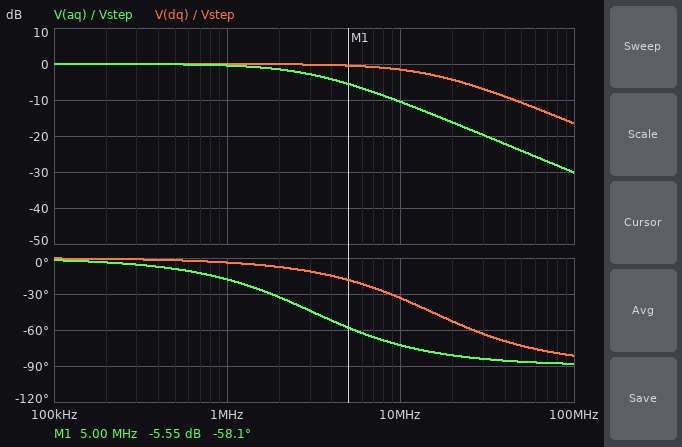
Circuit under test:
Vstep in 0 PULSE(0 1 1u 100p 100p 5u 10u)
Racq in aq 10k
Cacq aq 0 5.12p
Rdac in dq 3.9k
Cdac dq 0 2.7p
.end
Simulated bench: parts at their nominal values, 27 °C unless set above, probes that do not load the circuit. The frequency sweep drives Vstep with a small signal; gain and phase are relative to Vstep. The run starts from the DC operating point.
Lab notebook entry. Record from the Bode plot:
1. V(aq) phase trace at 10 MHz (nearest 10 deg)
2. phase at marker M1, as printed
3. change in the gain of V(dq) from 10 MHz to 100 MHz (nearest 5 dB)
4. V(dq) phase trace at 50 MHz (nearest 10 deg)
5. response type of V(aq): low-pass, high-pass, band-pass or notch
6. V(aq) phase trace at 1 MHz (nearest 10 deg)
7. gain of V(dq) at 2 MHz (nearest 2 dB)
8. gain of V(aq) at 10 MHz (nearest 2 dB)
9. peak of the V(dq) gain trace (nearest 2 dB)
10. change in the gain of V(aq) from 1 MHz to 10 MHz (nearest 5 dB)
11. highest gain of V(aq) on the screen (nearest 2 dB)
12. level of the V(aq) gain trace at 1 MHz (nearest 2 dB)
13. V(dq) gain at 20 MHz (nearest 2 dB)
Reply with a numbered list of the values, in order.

1. -70 deg
2. -58.1 deg
3. -15 dB
4. -70 deg
5. low-pass
6. -20 deg
7. 0 dB
8. -10 dB
9. 0 dB
10. -10 dB
11. 0 dB
12. 0 dB
13. -4 dB
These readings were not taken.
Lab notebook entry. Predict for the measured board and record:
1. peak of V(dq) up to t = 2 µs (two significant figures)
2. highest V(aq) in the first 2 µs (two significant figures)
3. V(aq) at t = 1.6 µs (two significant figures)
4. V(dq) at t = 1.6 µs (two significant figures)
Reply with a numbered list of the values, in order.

1. 1.0 V
2. 1.0 V
3. 1.0 V
4. 1.0 V
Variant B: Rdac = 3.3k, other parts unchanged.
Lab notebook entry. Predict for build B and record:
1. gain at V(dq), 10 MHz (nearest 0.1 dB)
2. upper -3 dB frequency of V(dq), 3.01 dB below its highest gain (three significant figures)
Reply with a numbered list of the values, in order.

1. -1.2 dB
2. 17.9 MHz
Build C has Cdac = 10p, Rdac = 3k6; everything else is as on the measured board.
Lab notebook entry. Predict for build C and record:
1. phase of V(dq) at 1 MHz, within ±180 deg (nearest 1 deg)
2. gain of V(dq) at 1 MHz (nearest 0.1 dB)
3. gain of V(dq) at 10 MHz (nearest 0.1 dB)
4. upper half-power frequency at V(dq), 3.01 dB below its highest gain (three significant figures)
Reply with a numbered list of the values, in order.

1. -13 deg
2. -0.2 dB
3. -7.9 dB
4. 4.42 MHz
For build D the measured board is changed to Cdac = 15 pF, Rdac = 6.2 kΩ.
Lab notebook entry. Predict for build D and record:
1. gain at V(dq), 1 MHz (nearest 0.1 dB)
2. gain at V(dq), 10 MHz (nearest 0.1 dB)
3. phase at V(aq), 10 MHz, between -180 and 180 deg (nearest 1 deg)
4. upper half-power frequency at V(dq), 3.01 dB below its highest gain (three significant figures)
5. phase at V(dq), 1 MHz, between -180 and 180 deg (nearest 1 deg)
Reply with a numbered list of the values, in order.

1. -1.3 dB
2. -15.5 dB
3. -73 deg
4. 1.71 MHz
5. -30 deg
